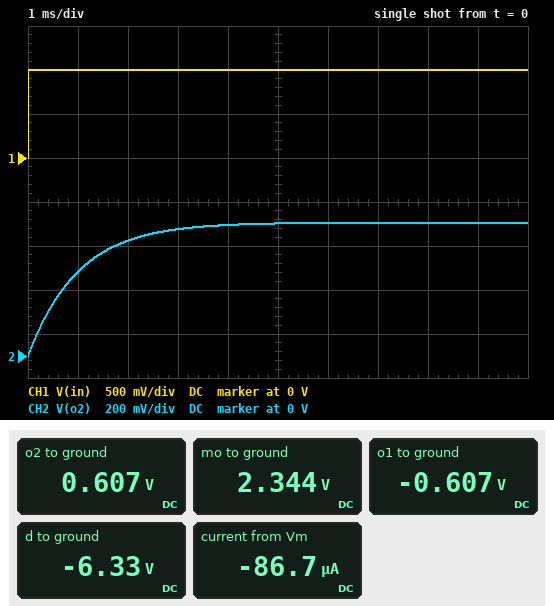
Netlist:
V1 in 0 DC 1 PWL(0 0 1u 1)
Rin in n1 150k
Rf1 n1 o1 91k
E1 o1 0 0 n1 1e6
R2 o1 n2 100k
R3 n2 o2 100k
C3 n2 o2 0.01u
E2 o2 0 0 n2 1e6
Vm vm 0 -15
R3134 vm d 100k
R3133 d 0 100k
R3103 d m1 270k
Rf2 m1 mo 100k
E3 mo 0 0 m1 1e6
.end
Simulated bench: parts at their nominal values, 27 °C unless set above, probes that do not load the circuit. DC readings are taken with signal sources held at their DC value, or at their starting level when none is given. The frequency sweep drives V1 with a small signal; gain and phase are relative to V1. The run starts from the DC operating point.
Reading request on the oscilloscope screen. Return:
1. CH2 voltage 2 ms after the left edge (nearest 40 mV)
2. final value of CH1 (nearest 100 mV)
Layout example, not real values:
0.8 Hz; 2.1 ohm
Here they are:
520 mV; 1.0 V
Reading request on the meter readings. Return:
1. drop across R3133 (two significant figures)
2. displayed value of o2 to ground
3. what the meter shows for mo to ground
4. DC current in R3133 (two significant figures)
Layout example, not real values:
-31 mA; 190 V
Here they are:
6.3 V; 0.607 V; 2.344 V; 63 µA
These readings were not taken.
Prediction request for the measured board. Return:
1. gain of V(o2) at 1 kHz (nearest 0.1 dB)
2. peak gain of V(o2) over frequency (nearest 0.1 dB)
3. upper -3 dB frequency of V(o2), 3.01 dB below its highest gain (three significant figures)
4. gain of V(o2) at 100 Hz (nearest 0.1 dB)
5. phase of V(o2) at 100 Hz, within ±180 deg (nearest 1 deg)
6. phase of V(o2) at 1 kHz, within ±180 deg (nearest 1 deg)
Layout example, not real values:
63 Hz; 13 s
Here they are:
-20.4 dB; -4.3 dB; 159 Hz; -5.8 dB; -32 deg; -81 deg
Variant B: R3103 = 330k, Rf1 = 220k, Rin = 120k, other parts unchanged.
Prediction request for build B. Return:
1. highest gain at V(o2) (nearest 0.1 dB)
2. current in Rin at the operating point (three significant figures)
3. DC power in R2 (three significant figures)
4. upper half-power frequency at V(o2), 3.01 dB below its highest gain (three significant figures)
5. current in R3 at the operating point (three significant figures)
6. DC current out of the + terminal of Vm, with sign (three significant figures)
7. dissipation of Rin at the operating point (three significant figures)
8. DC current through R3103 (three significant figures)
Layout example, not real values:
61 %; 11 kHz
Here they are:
5.3 dB; 8.33 µA; 33.6 µW; 159 Hz; 18.3 µA; -84.9 µA; 8.33 µW; 19.7 µA
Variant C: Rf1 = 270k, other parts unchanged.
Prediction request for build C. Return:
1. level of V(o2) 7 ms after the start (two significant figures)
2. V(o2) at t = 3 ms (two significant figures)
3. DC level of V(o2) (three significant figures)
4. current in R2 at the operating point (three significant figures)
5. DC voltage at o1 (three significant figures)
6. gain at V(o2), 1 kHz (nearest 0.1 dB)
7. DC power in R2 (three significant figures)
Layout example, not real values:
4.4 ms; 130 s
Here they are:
1.8 V; 1.7 V; 1.80 V; 18.0 µA; -1.80 V; -11.0 dB; 32.4 µW
